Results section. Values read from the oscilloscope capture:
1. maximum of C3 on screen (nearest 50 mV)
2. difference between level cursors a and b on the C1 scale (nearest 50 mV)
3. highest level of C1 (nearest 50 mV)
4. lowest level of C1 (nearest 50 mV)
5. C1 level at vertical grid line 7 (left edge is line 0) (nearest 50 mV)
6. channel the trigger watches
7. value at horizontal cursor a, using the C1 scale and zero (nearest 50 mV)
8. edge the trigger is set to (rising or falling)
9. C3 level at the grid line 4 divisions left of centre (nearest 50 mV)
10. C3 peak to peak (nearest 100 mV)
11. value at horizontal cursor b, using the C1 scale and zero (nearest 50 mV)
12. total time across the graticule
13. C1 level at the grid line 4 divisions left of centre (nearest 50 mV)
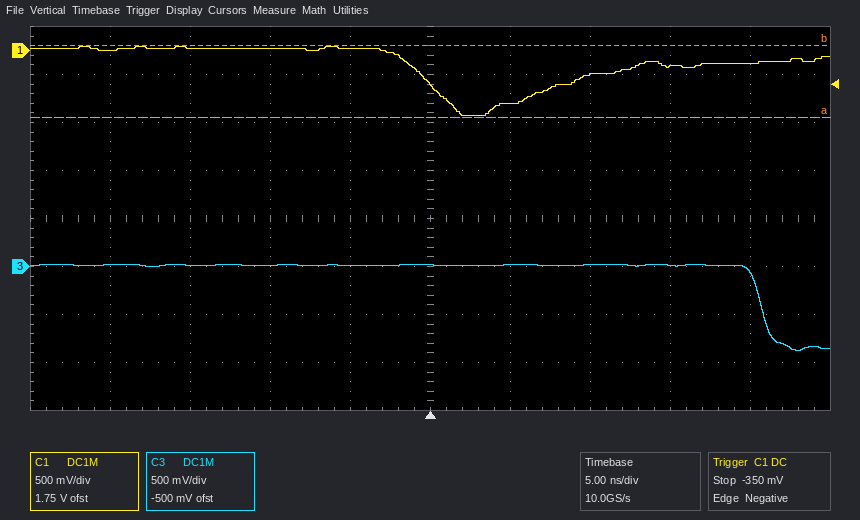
0 mV
750 mV
50 mV
-700 mV
-250 mV
C1
-700 mV
falling
0 mV
900 mV
50 mV
50 ns
0 mV
